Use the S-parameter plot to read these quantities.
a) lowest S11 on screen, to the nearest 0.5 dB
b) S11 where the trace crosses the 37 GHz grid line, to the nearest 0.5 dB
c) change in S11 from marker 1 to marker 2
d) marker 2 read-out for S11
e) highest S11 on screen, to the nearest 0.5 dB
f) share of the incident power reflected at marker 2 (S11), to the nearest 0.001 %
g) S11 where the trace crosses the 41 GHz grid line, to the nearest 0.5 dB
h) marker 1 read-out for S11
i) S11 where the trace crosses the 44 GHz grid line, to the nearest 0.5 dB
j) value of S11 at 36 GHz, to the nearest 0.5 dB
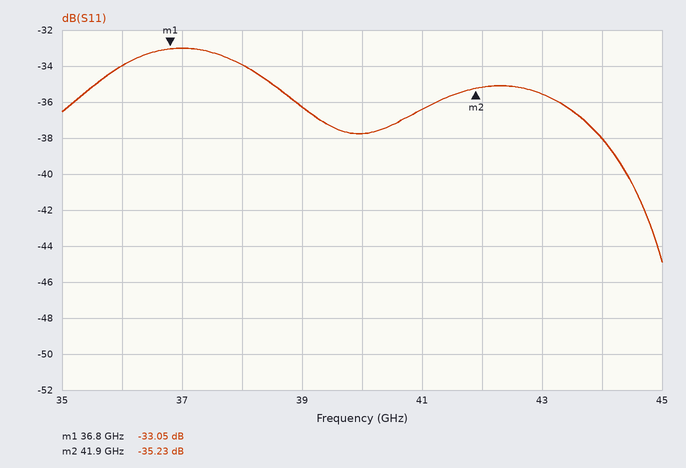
-45.0 dB
-33.0 dB
-2.18 dB
-35.23 dB
-33.0 dB
0.030 %
-36.5 dB
-33.05 dB
-38.0 dB
-34.0 dB
